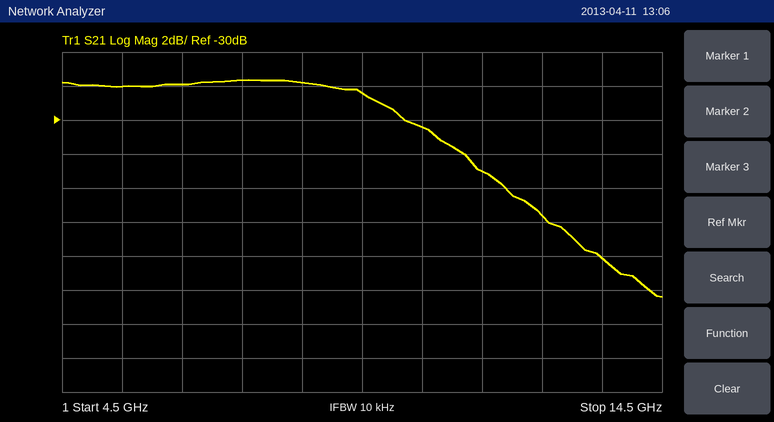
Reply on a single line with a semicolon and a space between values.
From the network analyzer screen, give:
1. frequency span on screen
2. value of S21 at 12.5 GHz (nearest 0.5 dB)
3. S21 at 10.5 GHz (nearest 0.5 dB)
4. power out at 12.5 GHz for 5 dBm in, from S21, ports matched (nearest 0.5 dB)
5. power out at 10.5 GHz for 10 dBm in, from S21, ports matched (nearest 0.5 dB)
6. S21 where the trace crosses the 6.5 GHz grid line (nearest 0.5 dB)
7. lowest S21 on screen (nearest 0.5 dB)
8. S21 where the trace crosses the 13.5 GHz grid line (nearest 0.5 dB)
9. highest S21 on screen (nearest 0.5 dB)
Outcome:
10 GHz; -35.5 dB; -30.5 dB; -30.5 dBm; -20.5 dBm; -28.0 dB; -40.5 dB; -38.0 dB; -27.5 dB
